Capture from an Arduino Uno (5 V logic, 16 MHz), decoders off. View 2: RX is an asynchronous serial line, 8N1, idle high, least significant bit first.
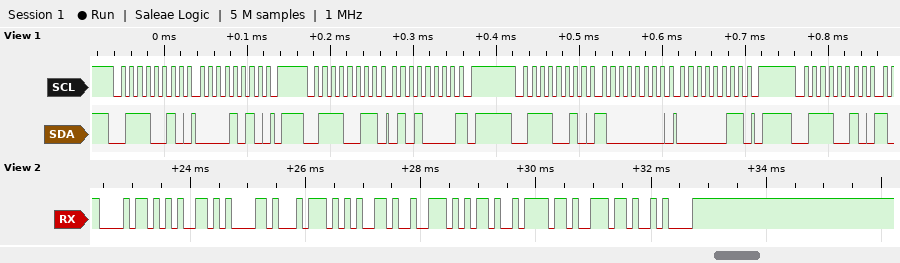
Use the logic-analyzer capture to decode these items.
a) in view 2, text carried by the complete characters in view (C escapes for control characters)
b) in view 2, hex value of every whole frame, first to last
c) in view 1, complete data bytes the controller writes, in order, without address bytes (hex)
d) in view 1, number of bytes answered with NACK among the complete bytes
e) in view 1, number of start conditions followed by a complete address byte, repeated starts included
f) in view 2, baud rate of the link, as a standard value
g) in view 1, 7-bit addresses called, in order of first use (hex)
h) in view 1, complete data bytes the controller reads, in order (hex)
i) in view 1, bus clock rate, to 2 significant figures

"heater-on\n"
0x68 0x65 0x61 0x74 0x65 0x72 0x2D 0x6F 0x6E 0x0A
0A 80 03
1
4
9600 baud
0x39
50
100 kHz
